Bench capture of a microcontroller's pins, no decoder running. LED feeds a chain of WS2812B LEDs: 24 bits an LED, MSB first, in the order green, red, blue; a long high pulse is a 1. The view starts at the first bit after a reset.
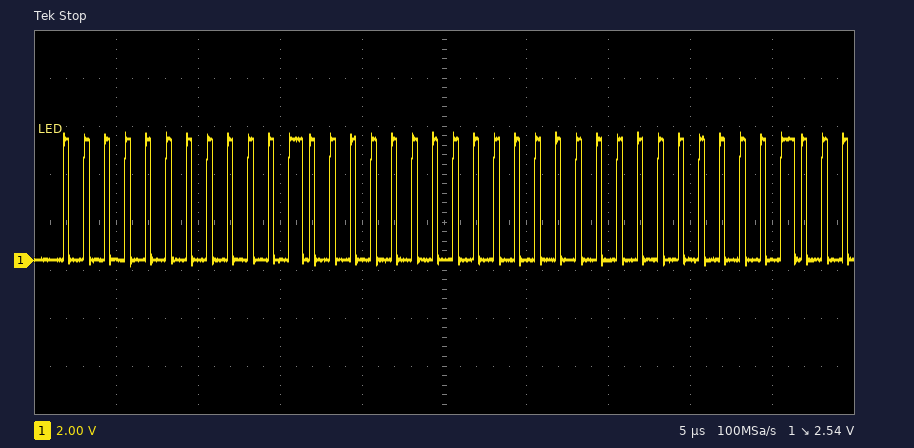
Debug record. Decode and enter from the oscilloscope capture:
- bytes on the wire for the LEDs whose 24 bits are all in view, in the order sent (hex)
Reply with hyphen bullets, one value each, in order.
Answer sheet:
- 00 10 00
